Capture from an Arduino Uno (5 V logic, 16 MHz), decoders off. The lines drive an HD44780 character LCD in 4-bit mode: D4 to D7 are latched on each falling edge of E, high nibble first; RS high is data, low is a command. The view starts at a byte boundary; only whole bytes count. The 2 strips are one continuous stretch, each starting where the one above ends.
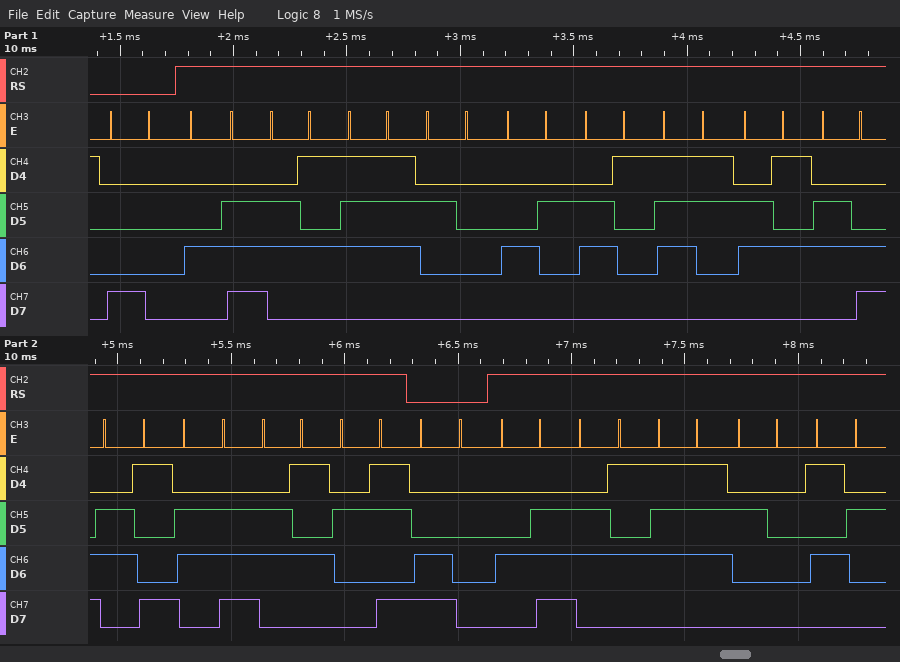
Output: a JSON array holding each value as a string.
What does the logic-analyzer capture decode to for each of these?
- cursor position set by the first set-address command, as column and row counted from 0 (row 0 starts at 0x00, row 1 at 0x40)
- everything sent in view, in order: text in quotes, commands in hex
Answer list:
["column 0, row 0", "0x80 \"New Baseline+\" 0xC0 \"New R\""]
